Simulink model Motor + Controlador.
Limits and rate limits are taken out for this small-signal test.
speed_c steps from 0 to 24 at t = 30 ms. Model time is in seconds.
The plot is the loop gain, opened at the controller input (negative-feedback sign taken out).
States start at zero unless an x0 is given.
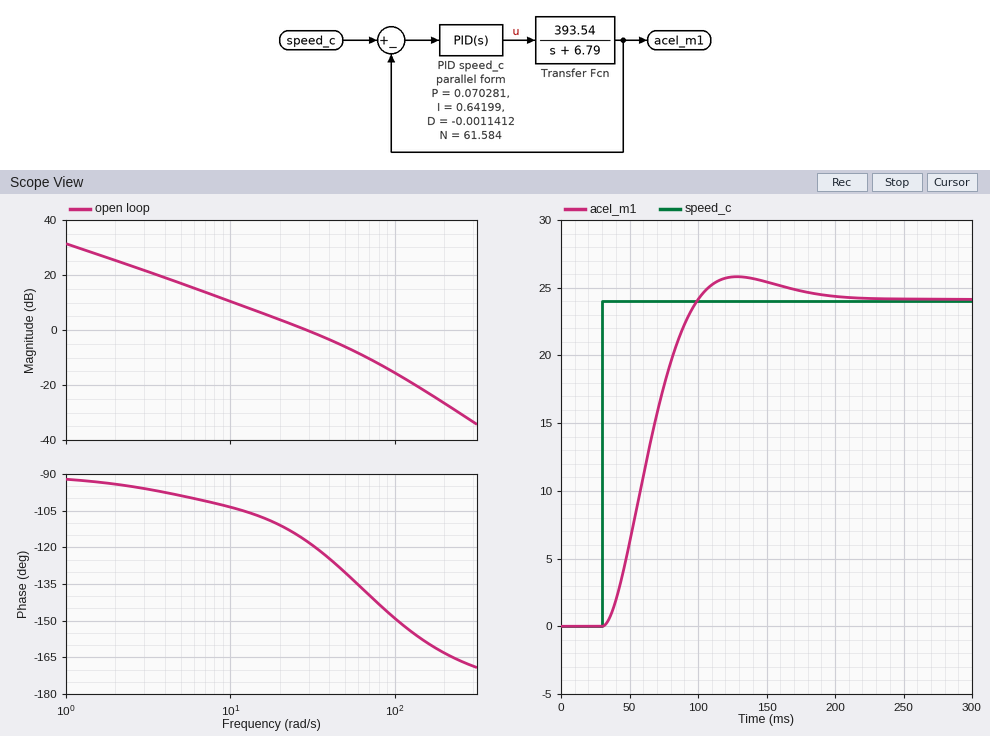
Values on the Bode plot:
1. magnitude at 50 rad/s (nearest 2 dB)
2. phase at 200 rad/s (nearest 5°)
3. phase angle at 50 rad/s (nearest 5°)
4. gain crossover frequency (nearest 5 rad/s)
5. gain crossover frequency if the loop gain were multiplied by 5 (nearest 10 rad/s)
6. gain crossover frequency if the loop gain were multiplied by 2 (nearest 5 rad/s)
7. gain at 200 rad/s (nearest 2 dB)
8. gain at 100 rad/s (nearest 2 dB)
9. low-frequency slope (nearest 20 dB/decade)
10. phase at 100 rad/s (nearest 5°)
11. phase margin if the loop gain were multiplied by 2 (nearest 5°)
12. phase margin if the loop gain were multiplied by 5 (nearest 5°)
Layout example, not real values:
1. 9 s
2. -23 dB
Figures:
1. -6 dB
2. -165°
3. -130°
4. 30 rad/s
5. 90 rad/s
6. 50 rad/s
7. -26 dB
8. -16 dB
9. -20 dB/decade
10. -150°
11. 50°
12. 35°
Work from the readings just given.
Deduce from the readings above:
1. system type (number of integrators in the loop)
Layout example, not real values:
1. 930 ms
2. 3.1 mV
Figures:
1. 1
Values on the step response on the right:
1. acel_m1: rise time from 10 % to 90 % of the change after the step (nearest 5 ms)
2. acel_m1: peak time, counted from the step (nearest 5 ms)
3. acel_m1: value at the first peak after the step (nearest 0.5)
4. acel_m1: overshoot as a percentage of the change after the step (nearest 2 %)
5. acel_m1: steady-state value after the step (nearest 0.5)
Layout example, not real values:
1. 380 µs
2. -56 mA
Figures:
1. 45 ms
2. 100 ms
3. 26.0
4. 8 %
5. 24.0
